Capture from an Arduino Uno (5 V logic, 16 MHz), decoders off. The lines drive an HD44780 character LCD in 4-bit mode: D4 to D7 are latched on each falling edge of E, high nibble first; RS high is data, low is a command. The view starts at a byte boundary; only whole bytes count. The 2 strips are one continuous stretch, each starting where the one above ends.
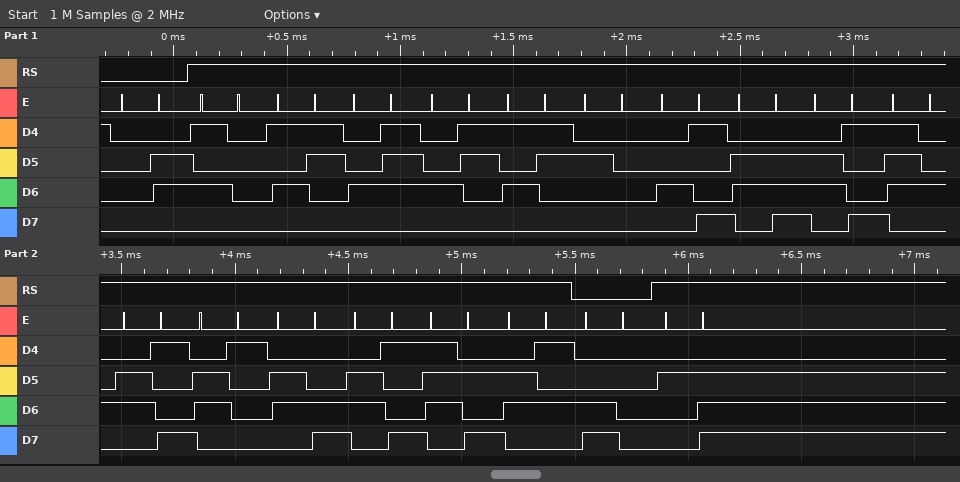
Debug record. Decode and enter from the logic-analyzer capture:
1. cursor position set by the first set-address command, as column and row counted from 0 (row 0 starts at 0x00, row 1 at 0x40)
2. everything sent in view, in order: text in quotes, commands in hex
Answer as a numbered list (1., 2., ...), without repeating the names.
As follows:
1. column 0, row 1
2. 0x06 "PSGCS Initialize" 0xC0 "."
